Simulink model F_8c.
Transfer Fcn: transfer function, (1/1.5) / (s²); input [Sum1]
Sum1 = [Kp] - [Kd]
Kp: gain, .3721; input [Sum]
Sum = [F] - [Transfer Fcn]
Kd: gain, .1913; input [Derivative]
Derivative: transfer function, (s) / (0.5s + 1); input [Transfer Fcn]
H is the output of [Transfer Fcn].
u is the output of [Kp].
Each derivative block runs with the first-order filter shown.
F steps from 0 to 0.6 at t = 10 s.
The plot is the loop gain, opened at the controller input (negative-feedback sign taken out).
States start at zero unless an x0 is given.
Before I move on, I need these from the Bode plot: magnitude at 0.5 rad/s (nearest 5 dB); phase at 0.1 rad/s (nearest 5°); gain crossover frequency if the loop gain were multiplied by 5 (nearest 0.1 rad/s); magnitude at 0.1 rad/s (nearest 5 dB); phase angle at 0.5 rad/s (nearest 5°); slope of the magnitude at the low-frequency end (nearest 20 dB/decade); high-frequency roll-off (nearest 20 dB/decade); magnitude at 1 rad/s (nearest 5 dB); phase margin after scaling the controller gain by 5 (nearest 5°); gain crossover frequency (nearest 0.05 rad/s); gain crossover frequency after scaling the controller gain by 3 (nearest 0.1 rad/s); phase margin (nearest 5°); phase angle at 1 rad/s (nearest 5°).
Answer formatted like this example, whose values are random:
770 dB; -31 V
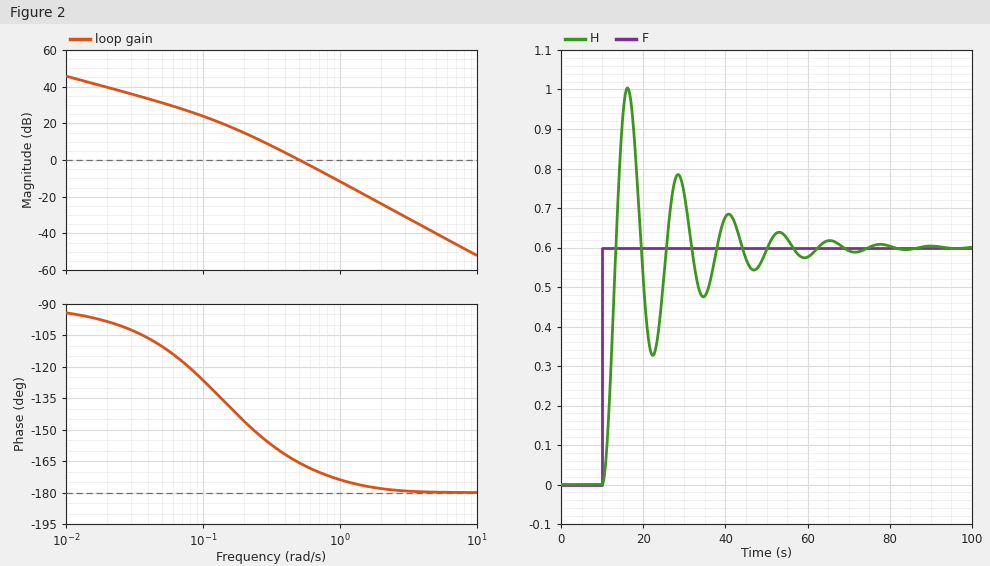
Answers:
0 dB; -125°; 1.1 rad/s; 25 dB; -165°; -20 dB/decade; -40 dB/decade; -10 dB; 5°; 0.50 rad/s; 0.9 rad/s; 15°; -175°
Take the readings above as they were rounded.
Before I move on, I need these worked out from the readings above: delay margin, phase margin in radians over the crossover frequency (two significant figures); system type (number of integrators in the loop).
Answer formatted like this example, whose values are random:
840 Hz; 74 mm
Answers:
0.52 s; 1
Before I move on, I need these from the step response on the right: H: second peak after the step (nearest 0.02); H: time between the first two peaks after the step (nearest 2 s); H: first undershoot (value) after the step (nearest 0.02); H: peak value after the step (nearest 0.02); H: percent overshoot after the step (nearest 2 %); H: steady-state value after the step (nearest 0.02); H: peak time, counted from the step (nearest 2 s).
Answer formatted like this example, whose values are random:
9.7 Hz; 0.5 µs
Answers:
0.78; 12 s; 0.32; 1.00; 68 %; 0.60; 6 s
